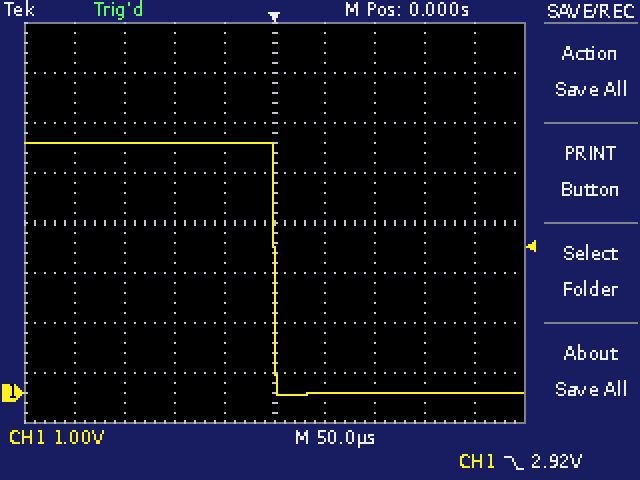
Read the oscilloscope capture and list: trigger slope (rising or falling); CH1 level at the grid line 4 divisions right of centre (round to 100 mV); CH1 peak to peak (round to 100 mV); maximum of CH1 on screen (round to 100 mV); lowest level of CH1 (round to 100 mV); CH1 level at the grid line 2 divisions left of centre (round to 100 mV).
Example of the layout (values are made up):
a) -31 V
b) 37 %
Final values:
a) falling
b) 0.0 V
c) 5.0 V
d) 5.0 V
e) 0.0 V
f) 5.0 V
